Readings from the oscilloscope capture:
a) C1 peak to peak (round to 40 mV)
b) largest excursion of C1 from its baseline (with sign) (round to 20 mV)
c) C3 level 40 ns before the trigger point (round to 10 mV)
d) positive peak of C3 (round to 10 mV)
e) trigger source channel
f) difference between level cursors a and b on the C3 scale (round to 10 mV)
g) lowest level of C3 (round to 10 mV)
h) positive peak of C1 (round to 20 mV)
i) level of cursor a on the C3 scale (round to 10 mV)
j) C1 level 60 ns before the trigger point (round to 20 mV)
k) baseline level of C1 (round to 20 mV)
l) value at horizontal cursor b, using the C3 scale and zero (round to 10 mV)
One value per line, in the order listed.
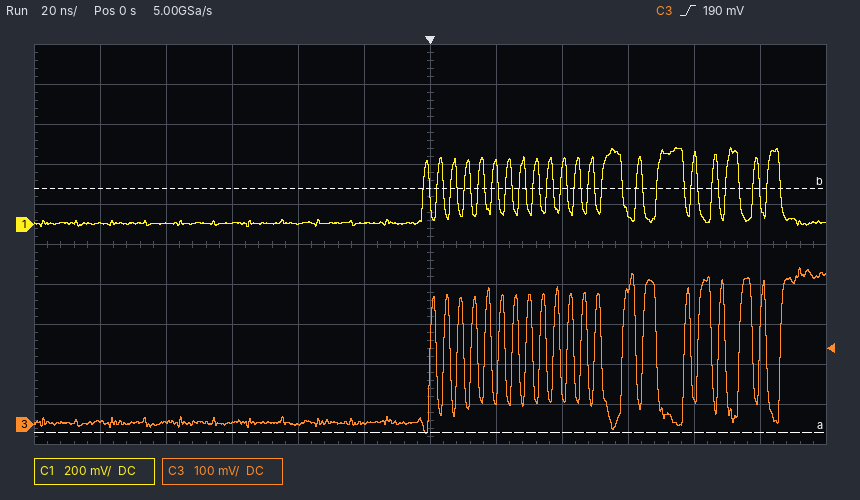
400 mV
+380 mV
0 mV
390 mV
C3
610 mV
-20 mV
380 mV
-20 mV
0 mV
0 mV
590 mV
